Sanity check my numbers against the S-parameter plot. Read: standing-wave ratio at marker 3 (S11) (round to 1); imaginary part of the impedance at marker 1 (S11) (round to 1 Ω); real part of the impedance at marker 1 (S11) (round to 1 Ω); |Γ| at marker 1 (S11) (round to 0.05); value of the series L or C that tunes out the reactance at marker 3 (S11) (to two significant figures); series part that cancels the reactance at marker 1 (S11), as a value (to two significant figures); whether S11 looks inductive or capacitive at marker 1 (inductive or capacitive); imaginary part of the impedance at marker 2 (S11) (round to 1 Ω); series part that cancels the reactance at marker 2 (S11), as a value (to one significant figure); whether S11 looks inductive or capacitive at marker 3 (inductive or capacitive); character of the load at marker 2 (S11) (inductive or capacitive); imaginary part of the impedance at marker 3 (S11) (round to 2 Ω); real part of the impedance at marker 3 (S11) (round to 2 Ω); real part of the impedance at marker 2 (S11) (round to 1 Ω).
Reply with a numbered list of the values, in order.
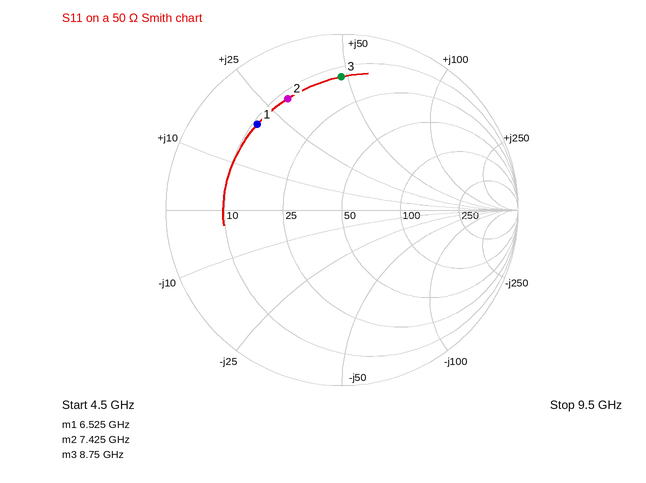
1. 7
2. +20 Ω
3. 11 Ω
4. 0.70
5. 380 fF
6. 1.2 pF
7. inductive
8. +30 Ω
9. 700 fF
10. inductive
11. inductive
12. +48 Ω
13. 14 Ω
14. 12 Ω
